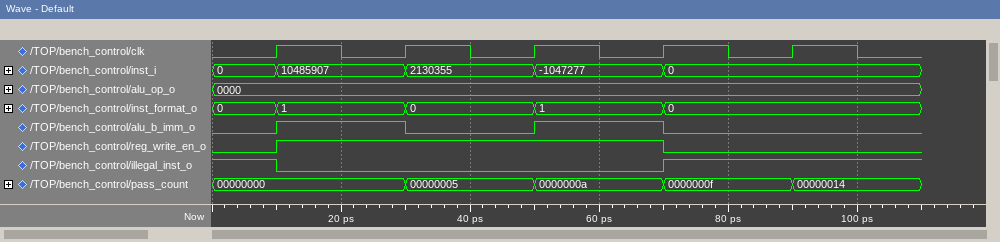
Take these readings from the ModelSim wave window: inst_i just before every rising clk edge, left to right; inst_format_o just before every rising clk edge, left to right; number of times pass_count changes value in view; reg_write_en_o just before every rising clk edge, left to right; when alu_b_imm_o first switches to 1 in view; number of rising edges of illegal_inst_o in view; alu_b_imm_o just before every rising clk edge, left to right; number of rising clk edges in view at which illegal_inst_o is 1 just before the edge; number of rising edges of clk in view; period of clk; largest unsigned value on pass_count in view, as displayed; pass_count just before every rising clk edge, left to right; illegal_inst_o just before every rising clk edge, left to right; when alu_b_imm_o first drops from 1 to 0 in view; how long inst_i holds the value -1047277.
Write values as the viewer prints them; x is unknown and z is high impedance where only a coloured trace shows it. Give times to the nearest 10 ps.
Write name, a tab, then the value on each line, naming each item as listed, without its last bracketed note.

inst_i just before every rising clk edge, left to right	0, 10485907, 2130355, -1047277, 0
inst_format_o just before every rising clk edge, left to right	0, 1, 0, 1, 0
number of times pass_count changes value in view	4
reg_write_en_o just before every rising clk edge, left to right	0 1 1 1 0
when alu_b_imm_o first switches to 1 in view	10 ps
number of rising edges of illegal_inst_o in view	1
alu_b_imm_o just before every rising clk edge, left to right	0 1 0 1 0
number of rising clk edges in view at which illegal_inst_o is 1 just before the edge	2
number of rising edges of clk in view	5
period of clk	20 ps
largest unsigned value on pass_count in view, as displayed	00000014
pass_count just before every rising clk edge, left to right	00000000, 00000000, 00000005, 0000000a, 0000000f
illegal_inst_o just before every rising clk edge, left to right	1 0 0 0 1
when alu_b_imm_o first drops from 1 to 0 in view	30 ps
how long inst_i holds the value -1047277	20 ps
